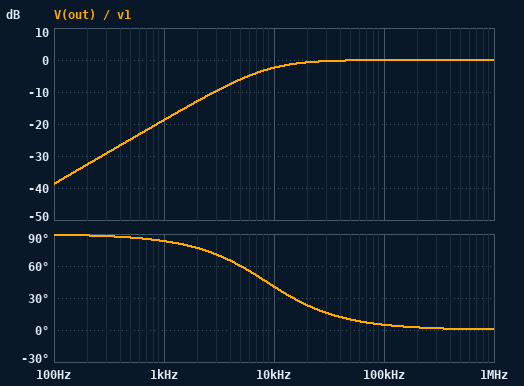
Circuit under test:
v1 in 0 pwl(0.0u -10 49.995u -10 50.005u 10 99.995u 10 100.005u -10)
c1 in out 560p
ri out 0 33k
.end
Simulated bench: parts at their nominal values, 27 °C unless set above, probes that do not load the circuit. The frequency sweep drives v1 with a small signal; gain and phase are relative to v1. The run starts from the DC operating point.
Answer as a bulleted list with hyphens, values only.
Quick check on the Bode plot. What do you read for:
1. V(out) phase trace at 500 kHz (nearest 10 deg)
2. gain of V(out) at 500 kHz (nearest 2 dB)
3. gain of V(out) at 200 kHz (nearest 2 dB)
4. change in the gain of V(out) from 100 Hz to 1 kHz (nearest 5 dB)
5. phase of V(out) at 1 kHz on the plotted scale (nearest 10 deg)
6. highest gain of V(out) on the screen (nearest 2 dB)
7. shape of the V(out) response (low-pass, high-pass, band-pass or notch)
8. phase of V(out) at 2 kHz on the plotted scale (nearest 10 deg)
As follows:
- 0 deg
- 0 dB
- 0 dB
- 20 dB
- 80 deg
- 0 dB
- high-pass
- 80 deg
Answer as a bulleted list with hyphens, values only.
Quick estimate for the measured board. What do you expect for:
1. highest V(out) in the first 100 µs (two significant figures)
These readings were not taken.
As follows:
- 20 V
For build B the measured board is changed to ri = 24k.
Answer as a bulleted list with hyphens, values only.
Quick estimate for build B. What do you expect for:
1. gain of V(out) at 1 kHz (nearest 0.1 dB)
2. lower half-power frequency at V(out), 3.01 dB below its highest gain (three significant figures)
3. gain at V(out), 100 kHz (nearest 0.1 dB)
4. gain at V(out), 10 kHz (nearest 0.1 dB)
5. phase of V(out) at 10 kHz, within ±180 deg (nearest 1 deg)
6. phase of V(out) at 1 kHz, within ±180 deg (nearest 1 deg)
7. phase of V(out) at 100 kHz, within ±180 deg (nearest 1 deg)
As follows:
- -21.5 dB
- 11.8 kHz
- -0.1 dB
- -3.8 dB
- 50 deg
- 85 deg
- 7 deg
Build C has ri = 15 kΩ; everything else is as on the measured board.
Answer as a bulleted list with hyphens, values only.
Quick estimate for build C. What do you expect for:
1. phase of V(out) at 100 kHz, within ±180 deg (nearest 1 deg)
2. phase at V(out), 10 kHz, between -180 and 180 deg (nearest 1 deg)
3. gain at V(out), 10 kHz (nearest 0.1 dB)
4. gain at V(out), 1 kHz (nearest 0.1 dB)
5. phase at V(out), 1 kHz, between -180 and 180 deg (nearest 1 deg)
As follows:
- 11 deg
- 62 deg
- -6.6 dB
- -25.6 dB
- 87 deg
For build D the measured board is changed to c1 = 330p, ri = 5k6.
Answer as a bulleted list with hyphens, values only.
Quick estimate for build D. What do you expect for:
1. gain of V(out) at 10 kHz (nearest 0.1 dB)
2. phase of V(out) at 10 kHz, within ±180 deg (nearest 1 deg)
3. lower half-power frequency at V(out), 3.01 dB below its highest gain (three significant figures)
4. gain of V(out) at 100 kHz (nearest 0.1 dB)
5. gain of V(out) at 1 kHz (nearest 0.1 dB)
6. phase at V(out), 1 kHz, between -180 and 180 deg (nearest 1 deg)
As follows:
- -18.8 dB
- 83 deg
- 86.1 kHz
- -2.4 dB
- -38.7 dB
- 89 deg
